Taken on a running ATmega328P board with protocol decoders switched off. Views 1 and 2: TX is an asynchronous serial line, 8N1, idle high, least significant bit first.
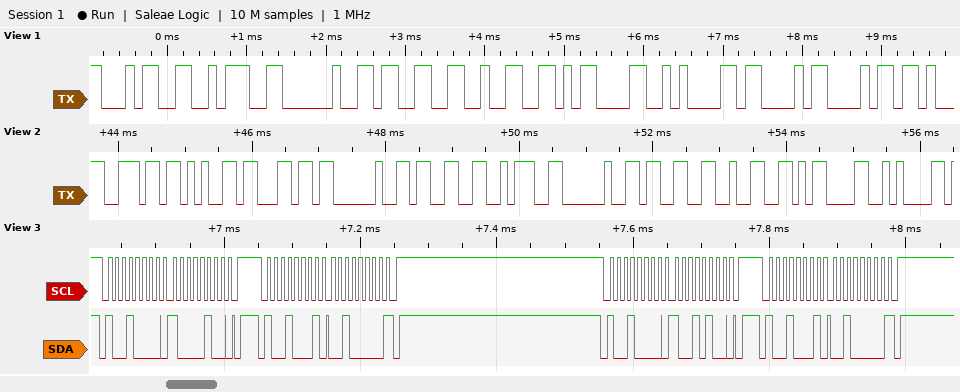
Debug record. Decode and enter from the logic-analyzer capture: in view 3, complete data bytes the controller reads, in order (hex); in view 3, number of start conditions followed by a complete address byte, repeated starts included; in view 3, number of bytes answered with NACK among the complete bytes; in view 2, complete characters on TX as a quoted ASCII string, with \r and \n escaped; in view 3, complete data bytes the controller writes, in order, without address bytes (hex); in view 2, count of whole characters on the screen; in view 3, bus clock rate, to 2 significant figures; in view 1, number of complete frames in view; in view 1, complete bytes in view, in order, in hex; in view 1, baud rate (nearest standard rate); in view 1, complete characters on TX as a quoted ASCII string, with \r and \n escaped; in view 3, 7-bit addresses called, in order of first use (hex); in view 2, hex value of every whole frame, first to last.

20 20
4
2
"nel 3: 32\r\n"
84 94
11
100 kHz
9
34 3A 20 33 32 0D 0A 43 68
9600 baud
"4: 32\r\nCh"
0x48
6E 65 6C 20 33 3A 20 33 32 0D 0A
